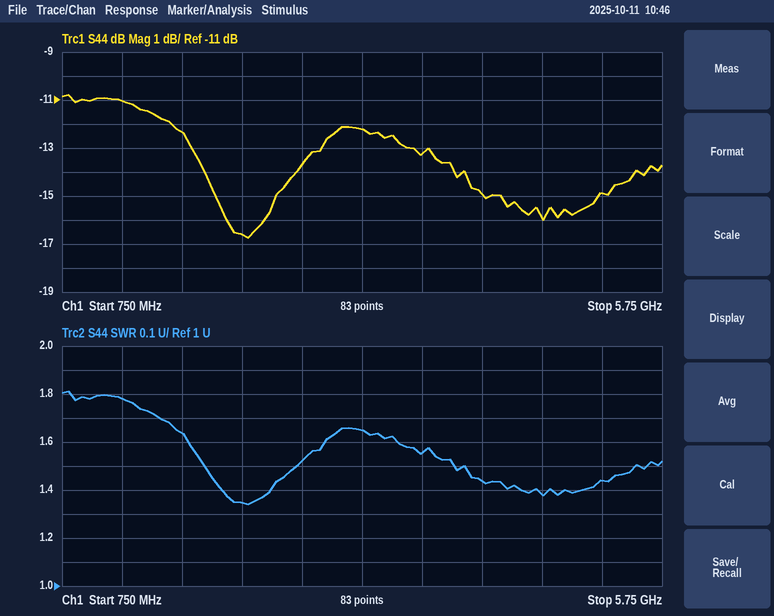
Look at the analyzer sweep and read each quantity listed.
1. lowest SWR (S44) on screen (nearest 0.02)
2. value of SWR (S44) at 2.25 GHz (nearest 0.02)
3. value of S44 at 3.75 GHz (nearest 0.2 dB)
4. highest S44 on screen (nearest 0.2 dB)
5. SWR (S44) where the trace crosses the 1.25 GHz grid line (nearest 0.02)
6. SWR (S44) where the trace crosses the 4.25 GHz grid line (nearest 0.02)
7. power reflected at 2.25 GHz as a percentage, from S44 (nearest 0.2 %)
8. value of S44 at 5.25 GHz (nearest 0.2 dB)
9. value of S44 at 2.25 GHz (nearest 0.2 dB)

1.34
1.34
-13.2 dB
-10.8 dB
1.78
1.44
2.2 %
-14.8 dB
-16.6 dB
